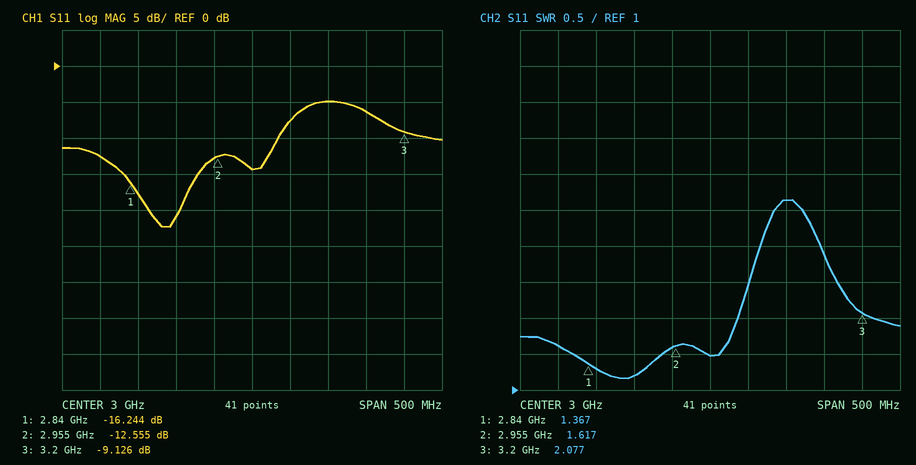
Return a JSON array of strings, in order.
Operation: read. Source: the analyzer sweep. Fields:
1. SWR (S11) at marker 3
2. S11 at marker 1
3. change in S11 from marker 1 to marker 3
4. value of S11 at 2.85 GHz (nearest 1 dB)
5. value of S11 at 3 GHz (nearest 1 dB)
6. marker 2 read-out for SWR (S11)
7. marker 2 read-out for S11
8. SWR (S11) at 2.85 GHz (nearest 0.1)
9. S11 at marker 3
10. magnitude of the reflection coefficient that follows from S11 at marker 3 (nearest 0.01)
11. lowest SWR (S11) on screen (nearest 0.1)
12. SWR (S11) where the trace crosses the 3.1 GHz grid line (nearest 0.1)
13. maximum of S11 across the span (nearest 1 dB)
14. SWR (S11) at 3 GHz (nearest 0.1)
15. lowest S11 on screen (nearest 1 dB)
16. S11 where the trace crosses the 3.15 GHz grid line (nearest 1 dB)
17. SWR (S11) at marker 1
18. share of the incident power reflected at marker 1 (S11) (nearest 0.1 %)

["2.077", "-16.244 dB", "7.118 dB", "-18 dB", "-14 dB", "1.617", "-12.555 dB", "1.3", "-9.126 dB", "0.35", "1.2", "3.6", "-5 dB", "1.5", "-22 dB", "-6 dB", "1.367", "2.4 %"]
